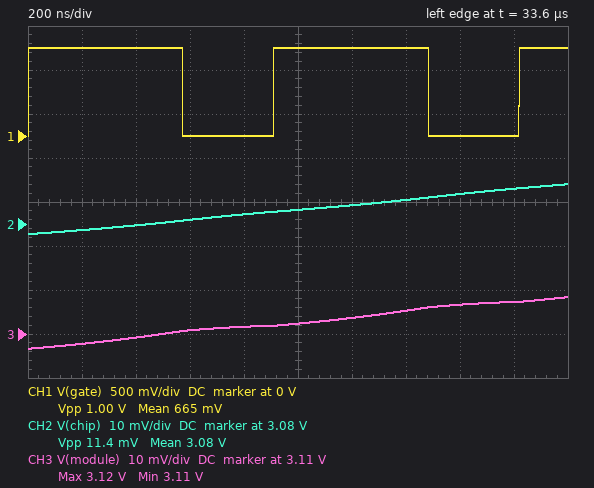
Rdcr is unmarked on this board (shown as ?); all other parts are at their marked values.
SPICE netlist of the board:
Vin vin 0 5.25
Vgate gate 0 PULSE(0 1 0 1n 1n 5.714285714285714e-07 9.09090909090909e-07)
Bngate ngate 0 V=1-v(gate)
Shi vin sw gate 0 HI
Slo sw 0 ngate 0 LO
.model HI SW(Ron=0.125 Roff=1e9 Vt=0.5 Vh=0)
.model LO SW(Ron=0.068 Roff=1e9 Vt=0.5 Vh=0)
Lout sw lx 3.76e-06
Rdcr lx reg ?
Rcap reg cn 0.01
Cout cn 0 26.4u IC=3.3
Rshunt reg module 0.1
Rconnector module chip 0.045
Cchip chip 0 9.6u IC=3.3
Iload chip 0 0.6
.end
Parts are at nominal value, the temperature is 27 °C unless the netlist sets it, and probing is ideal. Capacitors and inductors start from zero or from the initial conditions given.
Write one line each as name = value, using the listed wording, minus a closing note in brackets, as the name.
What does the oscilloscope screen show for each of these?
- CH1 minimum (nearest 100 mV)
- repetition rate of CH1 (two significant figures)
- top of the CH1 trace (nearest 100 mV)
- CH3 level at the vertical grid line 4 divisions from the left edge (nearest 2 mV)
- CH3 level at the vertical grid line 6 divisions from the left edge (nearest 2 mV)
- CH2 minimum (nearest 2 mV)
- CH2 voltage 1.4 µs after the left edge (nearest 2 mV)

CH1 minimum = 0 V
repetition rate of CH1 = 1.1 MHz
top of the CH1 trace = 1.0 V
CH3 level at the vertical grid line 4 divisions from the left edge = 3.112 V
CH3 level at the vertical grid line 6 divisions from the left edge = 3.114 V
CH2 minimum = 3.078 V
CH2 voltage 1.4 µs after the left edge = 3.086 V
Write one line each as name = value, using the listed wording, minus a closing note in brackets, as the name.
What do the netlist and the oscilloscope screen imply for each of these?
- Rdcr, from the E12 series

Rdcr, from the E12 series = 0.012 Ω
